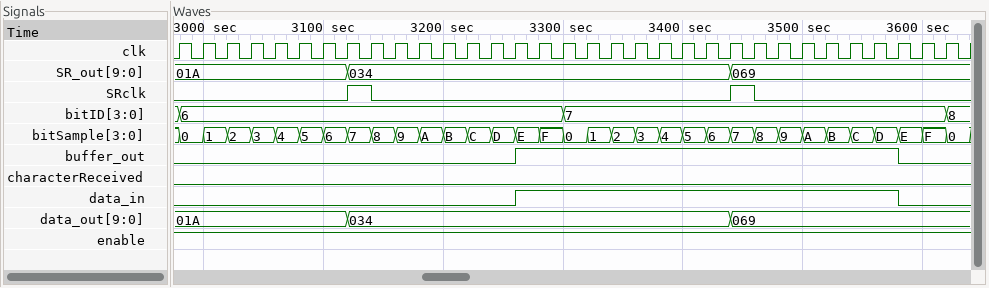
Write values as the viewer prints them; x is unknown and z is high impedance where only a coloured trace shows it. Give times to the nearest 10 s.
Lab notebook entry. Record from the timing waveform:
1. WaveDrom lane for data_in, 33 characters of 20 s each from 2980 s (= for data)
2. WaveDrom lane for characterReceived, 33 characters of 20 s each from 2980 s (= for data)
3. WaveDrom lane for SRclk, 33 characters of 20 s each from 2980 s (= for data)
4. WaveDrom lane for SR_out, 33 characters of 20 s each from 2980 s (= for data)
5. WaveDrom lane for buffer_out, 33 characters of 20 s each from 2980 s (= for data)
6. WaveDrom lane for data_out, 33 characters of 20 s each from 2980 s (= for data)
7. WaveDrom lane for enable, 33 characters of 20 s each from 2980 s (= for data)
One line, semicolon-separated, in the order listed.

{name: 'data_in', wave: '0.............1...............0..'}; {name: 'characterReceived', wave: '0................................'}; {name: 'SRclk', wave: '0......10..............10........'}; {name: 'SR_out', wave: '=......=...............=.........', data: '01A 034 069'}; {name: 'buffer_out', wave: '0.............1...............0..'}; {name: 'data_out', wave: '=......=...............=.........', data: '01A 034 069'}; {name: 'enable', wave: '1................................'}
